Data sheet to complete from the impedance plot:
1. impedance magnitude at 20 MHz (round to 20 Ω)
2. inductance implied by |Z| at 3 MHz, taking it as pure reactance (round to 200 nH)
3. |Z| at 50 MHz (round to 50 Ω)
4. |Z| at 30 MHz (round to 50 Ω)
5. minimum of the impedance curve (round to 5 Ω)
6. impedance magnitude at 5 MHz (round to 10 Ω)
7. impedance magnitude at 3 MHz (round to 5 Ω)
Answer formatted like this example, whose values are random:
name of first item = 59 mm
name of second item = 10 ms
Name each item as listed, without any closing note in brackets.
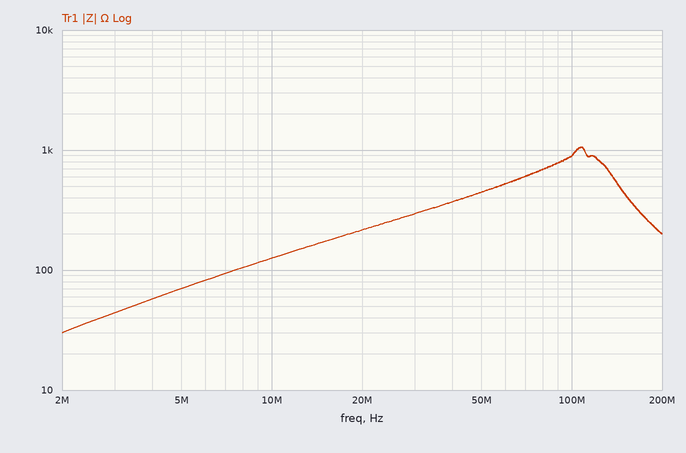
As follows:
impedance magnitude at 20 MHz = 220 Ω
inductance implied by |Z| at 3 MHz, taking it as pure reactance = 2.4 µH
|Z| at 50 MHz = 450 Ω
|Z| at 30 MHz = 300 Ω
minimum of the impedance curve = 30 Ω
impedance magnitude at 5 MHz = 70 Ω
impedance magnitude at 3 MHz = 45 Ω
